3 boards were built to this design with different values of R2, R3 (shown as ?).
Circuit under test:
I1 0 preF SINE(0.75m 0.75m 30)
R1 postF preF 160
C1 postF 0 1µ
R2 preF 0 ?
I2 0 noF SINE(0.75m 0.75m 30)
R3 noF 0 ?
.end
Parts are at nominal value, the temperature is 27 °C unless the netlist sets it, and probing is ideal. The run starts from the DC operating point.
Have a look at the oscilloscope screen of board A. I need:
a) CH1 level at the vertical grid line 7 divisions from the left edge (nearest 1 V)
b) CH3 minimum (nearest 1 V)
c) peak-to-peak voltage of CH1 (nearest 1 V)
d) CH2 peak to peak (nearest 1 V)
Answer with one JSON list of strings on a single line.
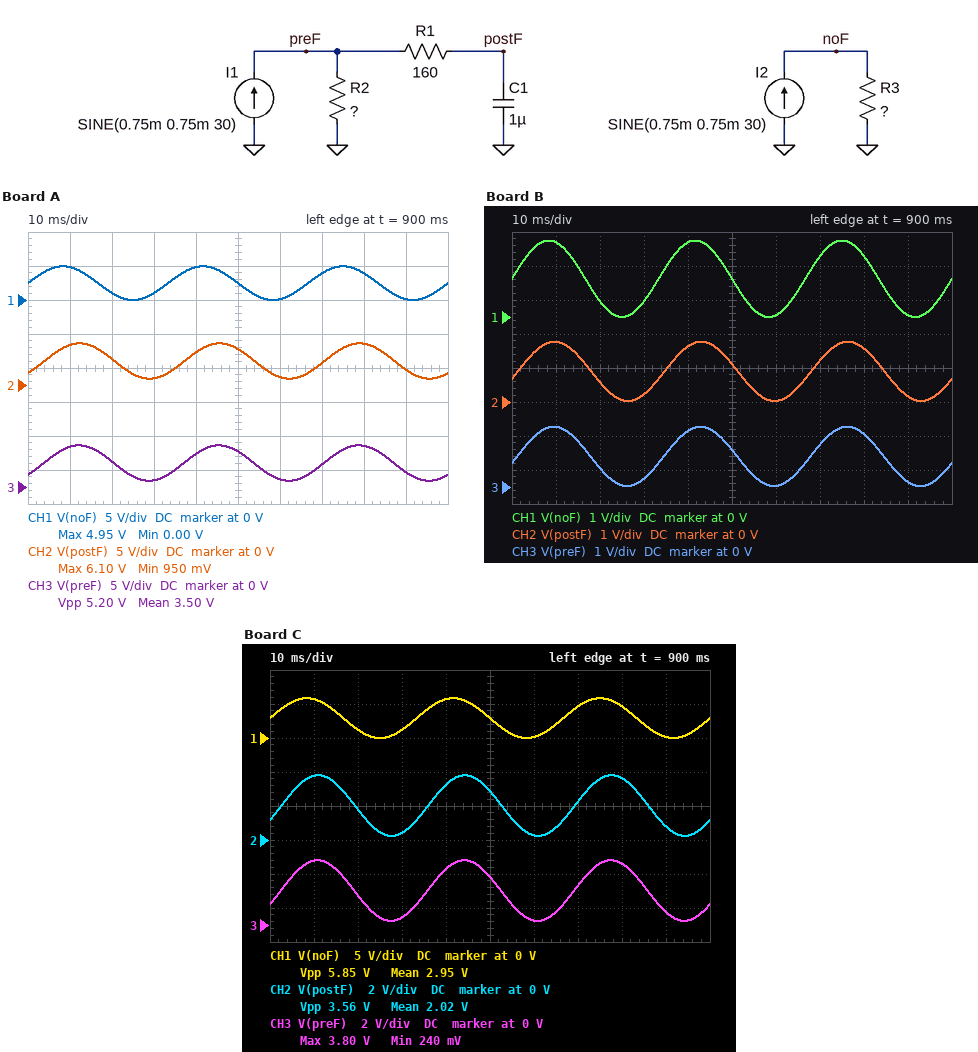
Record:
["4 V", "1 V", "5 V", "5 V"]
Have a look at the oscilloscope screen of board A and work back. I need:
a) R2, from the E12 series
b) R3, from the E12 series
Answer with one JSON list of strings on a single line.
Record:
["4.7 kΩ", "3.3 kΩ"]
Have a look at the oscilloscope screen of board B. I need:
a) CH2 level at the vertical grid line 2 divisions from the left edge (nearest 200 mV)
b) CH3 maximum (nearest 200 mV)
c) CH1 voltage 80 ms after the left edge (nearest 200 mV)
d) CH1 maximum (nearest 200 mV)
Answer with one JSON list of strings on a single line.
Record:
["600 mV", "1.8 V", "1.8 V", "2.2 V"]
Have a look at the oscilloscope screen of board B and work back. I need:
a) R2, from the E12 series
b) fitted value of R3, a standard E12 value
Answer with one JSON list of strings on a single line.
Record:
["1.2 kΩ", "1.5 kΩ"]
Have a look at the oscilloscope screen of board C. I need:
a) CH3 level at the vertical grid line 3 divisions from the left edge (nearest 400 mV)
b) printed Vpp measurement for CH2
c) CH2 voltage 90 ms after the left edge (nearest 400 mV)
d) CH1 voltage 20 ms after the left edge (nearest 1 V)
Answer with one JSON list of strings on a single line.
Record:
["400 mV", "3.56 V", "800 mV", "1 V"]
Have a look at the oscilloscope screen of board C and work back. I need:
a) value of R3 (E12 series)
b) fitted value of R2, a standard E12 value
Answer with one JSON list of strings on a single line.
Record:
["3.9 kΩ", "2.7 kΩ"]
